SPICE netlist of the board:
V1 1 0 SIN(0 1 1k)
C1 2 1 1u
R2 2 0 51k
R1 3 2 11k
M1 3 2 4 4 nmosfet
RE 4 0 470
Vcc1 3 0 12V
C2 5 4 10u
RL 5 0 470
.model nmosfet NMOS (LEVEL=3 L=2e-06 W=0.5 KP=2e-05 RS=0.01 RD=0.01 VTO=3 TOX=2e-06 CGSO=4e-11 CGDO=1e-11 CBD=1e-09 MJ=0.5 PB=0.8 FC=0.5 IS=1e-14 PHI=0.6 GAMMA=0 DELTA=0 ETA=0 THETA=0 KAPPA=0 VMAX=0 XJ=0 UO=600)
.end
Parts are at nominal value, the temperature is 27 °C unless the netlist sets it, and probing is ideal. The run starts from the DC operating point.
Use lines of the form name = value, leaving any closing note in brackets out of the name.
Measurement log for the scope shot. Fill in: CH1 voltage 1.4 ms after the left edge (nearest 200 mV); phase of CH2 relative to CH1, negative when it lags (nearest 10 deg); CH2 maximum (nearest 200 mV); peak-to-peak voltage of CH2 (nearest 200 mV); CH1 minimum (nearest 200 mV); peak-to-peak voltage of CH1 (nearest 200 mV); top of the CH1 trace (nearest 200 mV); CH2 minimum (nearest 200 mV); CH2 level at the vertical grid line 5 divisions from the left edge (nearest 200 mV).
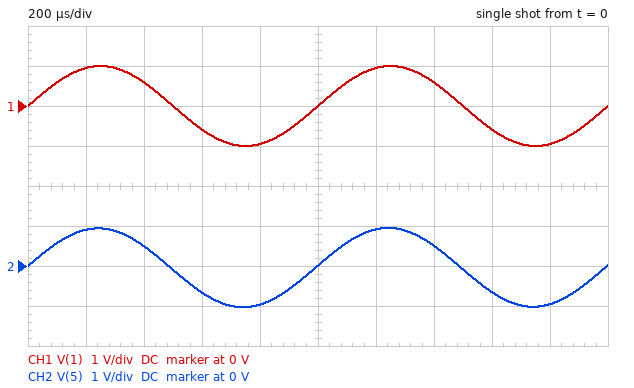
CH1 voltage 1.4 ms after the left edge = 600 mV
phase of CH2 relative to CH1, negative when it lags = 0 deg
CH2 maximum = 1.0 V
peak-to-peak voltage of CH2 = 2.0 V
CH1 minimum = -1.0 V
peak-to-peak voltage of CH1 = 2.0 V
top of the CH1 trace = 1.0 V
CH2 minimum = -1.0 V
CH2 level at the vertical grid line 5 divisions from the left edge = 0 V
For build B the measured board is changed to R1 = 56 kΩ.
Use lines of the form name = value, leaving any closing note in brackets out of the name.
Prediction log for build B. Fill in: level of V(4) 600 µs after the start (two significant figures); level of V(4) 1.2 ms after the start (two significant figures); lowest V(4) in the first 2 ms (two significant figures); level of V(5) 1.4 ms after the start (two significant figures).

level of V(4) 600 µs after the start = 2.1 V
level of V(4) 1.2 ms after the start = 3.6 V
lowest V(4) in the first 2 ms = 1.7 V
level of V(5) 1.4 ms after the start = 520 mV
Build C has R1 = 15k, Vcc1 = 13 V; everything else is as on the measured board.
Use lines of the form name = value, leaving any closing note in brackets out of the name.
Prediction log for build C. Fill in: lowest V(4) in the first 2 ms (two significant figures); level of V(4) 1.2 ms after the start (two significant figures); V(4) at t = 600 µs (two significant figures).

lowest V(4) in the first 2 ms = 6.0 V
level of V(4) 1.2 ms after the start = 7.9 V
V(4) at t = 600 µs = 6.4 V
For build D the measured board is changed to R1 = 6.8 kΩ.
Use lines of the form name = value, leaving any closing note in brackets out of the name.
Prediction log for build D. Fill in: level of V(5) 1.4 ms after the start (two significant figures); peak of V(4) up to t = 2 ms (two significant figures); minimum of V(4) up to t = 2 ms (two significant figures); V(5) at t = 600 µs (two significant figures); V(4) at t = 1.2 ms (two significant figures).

level of V(5) 1.4 ms after the start = 490 mV
peak of V(4) up to t = 2 ms = 8.5 V
minimum of V(4) up to t = 2 ms = 6.5 V
V(5) at t = 600 µs = -680 mV
V(4) at t = 1.2 ms = 8.4 V
